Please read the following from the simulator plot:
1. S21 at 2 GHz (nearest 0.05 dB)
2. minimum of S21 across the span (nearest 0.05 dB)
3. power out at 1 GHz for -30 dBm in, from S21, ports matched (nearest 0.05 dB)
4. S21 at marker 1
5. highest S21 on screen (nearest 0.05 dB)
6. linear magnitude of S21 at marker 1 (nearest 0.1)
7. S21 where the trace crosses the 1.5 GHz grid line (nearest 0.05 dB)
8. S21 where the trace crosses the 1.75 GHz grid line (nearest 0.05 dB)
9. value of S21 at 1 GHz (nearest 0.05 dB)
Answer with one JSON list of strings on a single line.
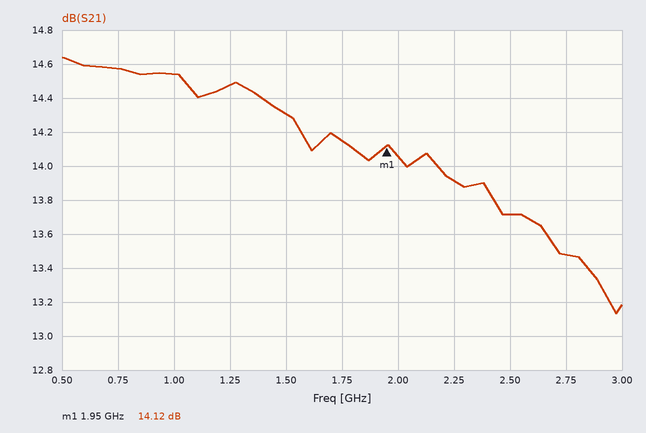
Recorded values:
["14.05 dB", "13.15 dB", "-15.45 dBm", "14.12 dB", "14.65 dB", "5.1", "14.30 dB", "14.15 dB", "14.55 dB"]
